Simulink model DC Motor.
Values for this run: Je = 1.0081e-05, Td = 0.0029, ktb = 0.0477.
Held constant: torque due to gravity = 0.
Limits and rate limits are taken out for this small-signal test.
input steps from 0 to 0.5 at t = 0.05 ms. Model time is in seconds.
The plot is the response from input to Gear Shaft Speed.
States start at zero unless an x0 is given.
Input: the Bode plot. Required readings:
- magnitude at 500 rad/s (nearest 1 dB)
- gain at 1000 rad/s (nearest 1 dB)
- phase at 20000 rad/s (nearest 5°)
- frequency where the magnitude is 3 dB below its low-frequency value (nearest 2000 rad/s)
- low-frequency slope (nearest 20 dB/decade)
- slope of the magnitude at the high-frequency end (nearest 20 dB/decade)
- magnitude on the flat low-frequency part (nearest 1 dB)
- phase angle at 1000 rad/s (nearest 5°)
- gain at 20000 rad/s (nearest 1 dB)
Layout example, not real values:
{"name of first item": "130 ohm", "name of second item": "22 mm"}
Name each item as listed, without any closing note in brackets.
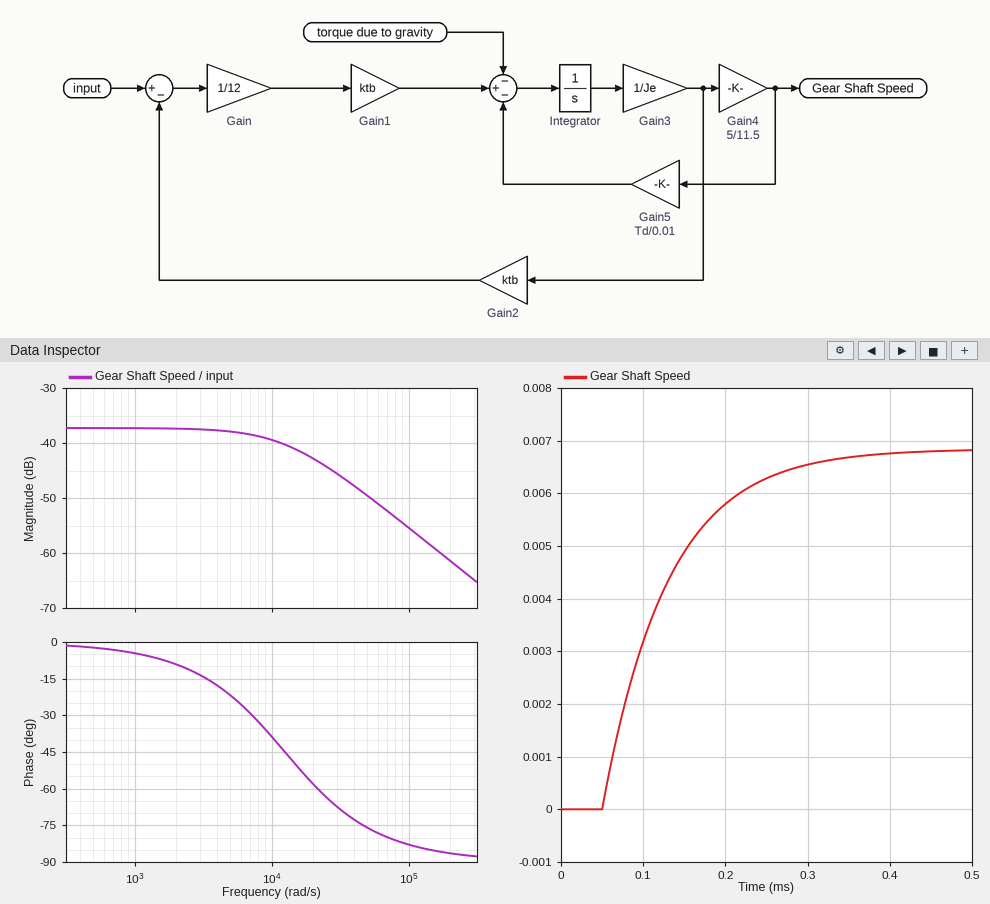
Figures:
{"magnitude at 500 rad/s": "-37 dB", "gain at 1000 rad/s": "-37 dB", "phase at 20000 rad/s": "-60°", "frequency where the magnitude is 3 dB below its low-frequency value": "12000 rad/s", "low-frequency slope": "0 dB/decade", "slope of the magnitude at the high-frequency end": "-20 dB/decade", "magnitude on the flat low-frequency part": "-37 dB", "phase angle at 1000 rad/s": "-5°", "gain at 20000 rad/s": "-43 dB"}
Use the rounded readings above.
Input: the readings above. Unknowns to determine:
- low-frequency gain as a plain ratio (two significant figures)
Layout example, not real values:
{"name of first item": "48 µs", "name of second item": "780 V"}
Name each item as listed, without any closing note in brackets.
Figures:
{"low-frequency gain as a plain ratio": "0.014"}
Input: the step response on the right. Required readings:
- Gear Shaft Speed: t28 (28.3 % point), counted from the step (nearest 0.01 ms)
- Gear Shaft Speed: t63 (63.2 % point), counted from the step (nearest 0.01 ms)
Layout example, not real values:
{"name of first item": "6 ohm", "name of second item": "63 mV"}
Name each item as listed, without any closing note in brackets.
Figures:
{"Gear Shaft Speed: t28 (28.3 % point), counted from the step": "0.03 ms", "Gear Shaft Speed: t63 (63.2 % point), counted from the step": "0.08 ms"}
